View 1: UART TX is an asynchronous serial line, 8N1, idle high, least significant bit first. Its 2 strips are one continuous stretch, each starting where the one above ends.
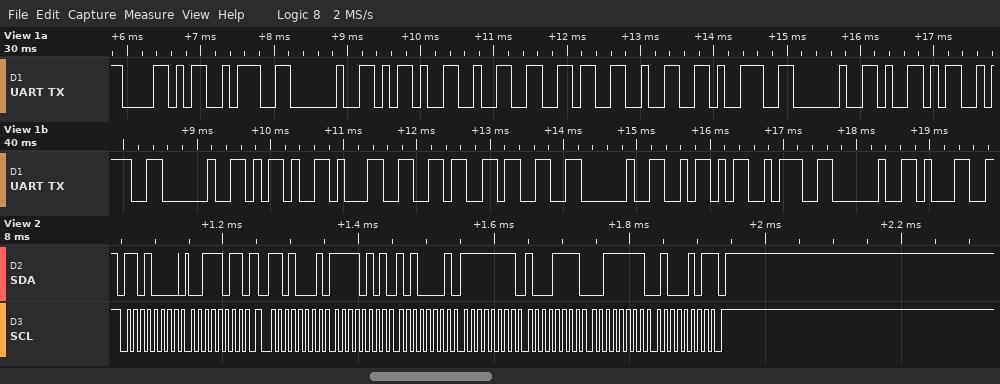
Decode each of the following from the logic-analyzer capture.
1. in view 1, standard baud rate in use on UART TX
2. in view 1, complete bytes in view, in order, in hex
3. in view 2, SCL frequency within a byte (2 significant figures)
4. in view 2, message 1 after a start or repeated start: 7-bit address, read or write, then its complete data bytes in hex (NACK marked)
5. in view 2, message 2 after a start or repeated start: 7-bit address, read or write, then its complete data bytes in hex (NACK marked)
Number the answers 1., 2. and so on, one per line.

1. 9600 baud
2. 0x58 0x3A 0x20 0x2D 0x32 0x36 0x32 0x39 0x20 0x59 0x3A 0x20 0x2D 0x31 0x36 0x33 0x20 0x5A 0x3A 0x20 0x31
3. 100 kHz
4. 0x68 write: 3B
5. 0x68 read: F5 A1 FF 8F 3F 45 NACK
